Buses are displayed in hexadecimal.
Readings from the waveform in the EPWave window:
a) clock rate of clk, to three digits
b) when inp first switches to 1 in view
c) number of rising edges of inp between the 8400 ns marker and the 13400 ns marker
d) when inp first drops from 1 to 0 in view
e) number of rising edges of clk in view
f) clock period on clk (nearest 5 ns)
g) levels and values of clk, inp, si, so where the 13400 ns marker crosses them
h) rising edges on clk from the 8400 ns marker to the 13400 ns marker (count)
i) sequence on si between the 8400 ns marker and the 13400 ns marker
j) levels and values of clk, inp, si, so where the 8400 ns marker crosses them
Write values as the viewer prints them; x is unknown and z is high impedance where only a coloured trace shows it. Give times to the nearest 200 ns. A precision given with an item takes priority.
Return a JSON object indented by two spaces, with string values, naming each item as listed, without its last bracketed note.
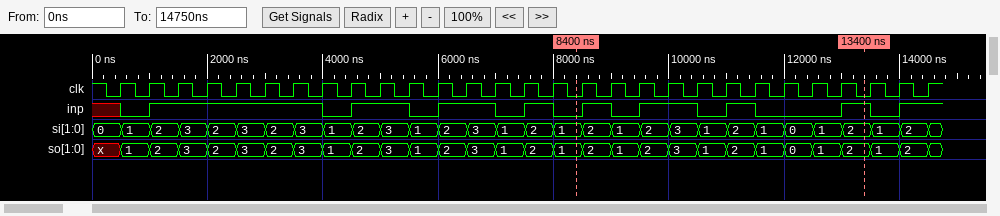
{
  "clock rate of clk, to three digits": "2.00 MHz",
  "when inp first switches to 1 in view": "1000 ns",
  "number of rising edges of inp between the 8400 ns marker and the 13400 ns marker": "4",
  "when inp first drops from 1 to 0 in view": "4000 ns",
  "number of rising edges of clk in view": "29",
  "clock period on clk": "500 ns",
  "levels and values of clk, inp, si, so where the 13400 ns marker crosses them": "clk=0, inp=1, si=2, so=2",
  "rising edges on clk from the 8400 ns marker to the 13400 ns marker": "10",
  "sequence on si between the 8400 ns marker and the 13400 ns marker": "1, 2, 1, 2, 3, 1, 2, 1, 0, 1, 2",
  "levels and values of clk, inp, si, so where the 8400 ns marker crosses them": "clk=0, inp=0, si=1, so=1"
}
